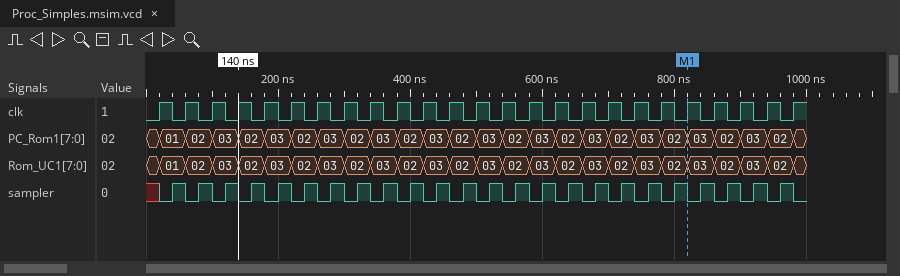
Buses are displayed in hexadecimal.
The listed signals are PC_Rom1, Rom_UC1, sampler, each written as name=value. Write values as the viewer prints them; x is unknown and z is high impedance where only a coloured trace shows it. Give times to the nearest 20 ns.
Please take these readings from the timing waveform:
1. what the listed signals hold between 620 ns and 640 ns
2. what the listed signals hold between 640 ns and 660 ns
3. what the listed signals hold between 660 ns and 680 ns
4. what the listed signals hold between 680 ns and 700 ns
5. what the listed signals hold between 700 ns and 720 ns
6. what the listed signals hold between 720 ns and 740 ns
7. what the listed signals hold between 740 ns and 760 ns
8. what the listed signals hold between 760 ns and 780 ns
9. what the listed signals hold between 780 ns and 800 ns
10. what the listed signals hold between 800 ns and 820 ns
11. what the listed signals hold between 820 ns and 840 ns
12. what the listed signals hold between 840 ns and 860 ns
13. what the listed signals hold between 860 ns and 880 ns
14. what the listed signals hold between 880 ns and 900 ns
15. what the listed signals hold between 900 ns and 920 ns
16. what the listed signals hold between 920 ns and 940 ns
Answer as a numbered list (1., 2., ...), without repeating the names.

1. PC_Rom1=02, Rom_UC1=02, sampler=0
2. PC_Rom1=02, Rom_UC1=02, sampler=1
3. PC_Rom1=03, Rom_UC1=03, sampler=0
4. PC_Rom1=03, Rom_UC1=03, sampler=1
5. PC_Rom1=02, Rom_UC1=02, sampler=0
6. PC_Rom1=02, Rom_UC1=02, sampler=1
7. PC_Rom1=03, Rom_UC1=03, sampler=0
8. PC_Rom1=03, Rom_UC1=03, sampler=1
9. PC_Rom1=02, Rom_UC1=02, sampler=0
10. PC_Rom1=02, Rom_UC1=02, sampler=1
11. PC_Rom1=03, Rom_UC1=03, sampler=0
12. PC_Rom1=03, Rom_UC1=03, sampler=1
13. PC_Rom1=02, Rom_UC1=02, sampler=0
14. PC_Rom1=02, Rom_UC1=02, sampler=1
15. PC_Rom1=03, Rom_UC1=03, sampler=0
16. PC_Rom1=03, Rom_UC1=03, sampler=1
